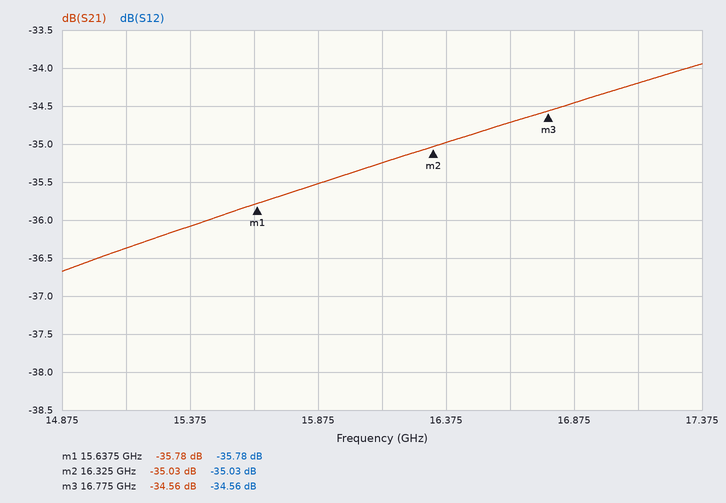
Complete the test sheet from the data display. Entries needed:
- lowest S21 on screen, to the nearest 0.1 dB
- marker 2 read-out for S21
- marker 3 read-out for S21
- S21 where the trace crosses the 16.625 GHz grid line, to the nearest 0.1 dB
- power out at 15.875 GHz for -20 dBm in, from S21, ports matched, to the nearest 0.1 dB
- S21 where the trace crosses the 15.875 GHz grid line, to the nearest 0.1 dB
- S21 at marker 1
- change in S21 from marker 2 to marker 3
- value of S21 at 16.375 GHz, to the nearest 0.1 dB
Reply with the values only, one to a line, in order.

-36.7 dB
-35.03 dB
-34.56 dB
-34.7 dB
-55.5 dBm
-35.5 dB
-35.78 dB
0.47 dB
-35.0 dB
